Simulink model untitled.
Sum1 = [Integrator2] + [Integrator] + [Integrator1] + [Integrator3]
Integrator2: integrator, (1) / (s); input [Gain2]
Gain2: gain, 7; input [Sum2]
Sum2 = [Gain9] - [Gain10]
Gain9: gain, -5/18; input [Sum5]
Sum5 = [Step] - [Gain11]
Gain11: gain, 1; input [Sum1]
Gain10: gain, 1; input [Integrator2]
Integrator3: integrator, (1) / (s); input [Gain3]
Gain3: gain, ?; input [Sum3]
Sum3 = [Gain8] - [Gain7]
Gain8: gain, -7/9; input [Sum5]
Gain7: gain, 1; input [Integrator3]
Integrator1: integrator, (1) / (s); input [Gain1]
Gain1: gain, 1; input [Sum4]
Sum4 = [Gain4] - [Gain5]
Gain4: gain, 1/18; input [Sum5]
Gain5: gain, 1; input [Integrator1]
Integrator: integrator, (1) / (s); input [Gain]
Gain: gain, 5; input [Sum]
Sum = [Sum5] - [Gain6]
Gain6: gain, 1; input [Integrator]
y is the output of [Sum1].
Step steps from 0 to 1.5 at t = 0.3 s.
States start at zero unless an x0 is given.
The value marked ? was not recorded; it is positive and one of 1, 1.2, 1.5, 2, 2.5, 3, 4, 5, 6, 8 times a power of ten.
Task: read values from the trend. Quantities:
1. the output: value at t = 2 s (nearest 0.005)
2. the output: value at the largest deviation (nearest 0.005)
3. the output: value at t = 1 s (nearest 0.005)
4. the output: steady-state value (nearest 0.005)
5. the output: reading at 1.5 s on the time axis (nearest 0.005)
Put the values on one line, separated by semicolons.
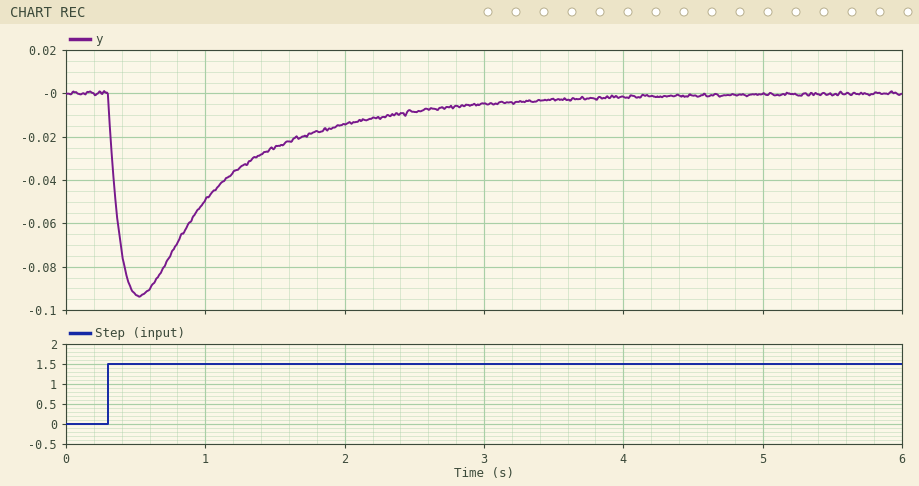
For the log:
-0.015; -0.095; -0.050; 0.000; -0.025
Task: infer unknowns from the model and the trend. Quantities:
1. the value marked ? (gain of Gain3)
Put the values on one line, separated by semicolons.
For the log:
5
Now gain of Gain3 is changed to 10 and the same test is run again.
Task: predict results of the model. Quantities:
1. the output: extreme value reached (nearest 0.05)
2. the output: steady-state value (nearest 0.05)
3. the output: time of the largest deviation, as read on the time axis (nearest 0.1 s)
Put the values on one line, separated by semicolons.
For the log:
-0.50; 0.00; 0.5 s
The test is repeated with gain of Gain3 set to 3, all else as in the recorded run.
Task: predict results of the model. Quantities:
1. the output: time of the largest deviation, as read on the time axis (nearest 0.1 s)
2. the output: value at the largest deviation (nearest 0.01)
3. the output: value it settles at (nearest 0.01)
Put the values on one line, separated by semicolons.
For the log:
0.6 s; 0.12; 0.00
